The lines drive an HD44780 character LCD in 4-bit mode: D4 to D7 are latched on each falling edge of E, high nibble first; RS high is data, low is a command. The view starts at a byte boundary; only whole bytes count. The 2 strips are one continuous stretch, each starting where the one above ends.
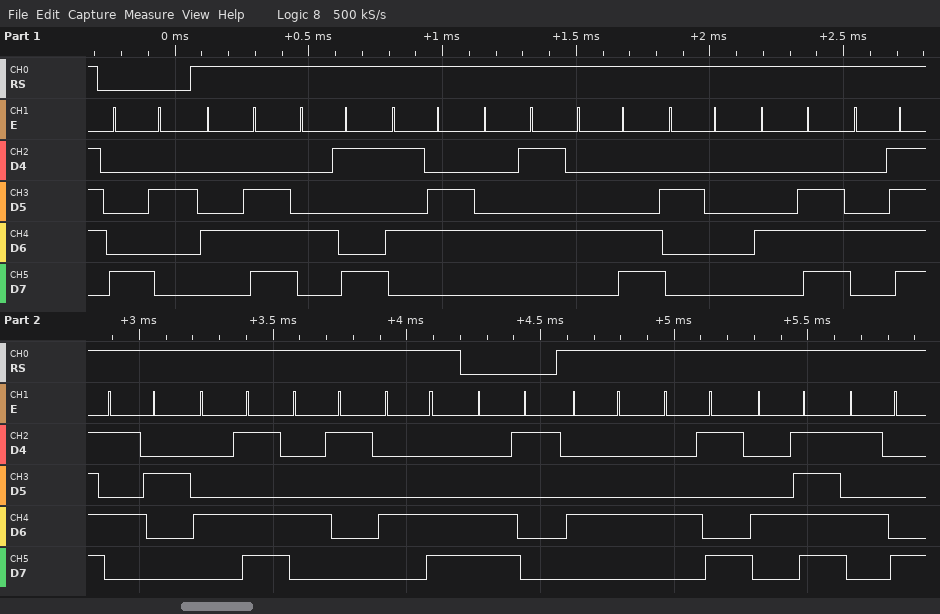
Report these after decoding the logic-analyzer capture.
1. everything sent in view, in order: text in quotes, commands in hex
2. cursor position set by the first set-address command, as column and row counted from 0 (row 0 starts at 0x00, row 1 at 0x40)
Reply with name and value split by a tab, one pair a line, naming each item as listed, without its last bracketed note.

everything sent in view, in order: text in quotes, commands in hex	0x82 "NIVEL NORMAL" 0xC1 "DIOX"
cursor position set by the first set-address command, as column and row counted from 0	column 2, row 0
